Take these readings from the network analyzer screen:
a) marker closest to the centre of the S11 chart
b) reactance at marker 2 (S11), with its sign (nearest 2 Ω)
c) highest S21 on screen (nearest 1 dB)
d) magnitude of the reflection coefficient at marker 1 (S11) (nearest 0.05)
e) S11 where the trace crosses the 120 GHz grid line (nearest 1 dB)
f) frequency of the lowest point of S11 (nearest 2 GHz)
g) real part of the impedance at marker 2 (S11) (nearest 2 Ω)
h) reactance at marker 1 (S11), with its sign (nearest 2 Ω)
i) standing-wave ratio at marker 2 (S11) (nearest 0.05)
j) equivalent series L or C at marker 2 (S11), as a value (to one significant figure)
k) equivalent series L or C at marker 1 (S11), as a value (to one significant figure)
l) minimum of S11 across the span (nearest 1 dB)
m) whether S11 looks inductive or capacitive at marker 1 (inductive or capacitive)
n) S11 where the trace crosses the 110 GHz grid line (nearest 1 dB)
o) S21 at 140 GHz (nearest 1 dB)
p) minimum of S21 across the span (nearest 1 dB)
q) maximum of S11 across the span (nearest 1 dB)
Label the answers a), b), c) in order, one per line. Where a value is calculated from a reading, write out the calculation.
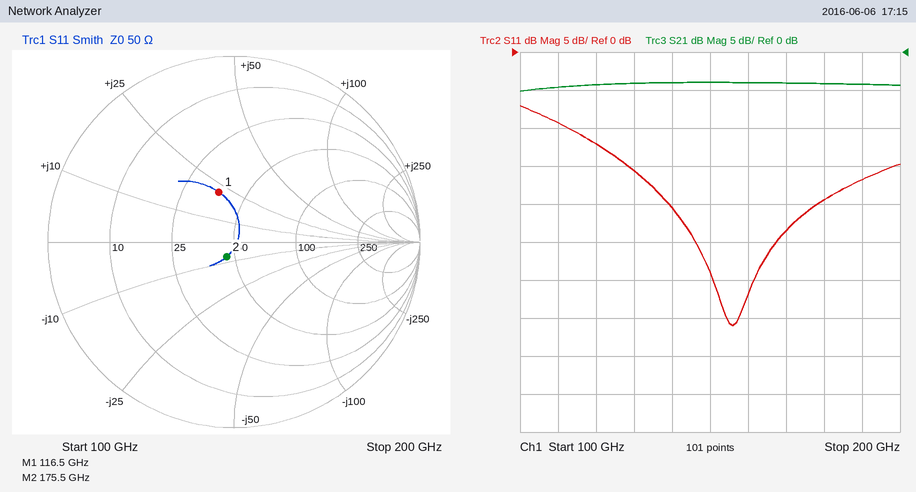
a) marker 2
b) -8 Ω
c) -4 dB
d) 0.30
e) -12 dB
f) 156 GHz
g) 46 Ω
h) +22 Ω
i) 1.20
j) C = 1/(2π × 175.5 GHz × 8 Ω) ≈ 113 fF, so 100 fF to one significant figure
k) L = 22 Ω/(2π × 116.5 GHz) ≈ 30 pH
l) -36 dB
m) inductive
n) -9 dB
o) -4 dB
p) -5 dB
q) -7 dB
